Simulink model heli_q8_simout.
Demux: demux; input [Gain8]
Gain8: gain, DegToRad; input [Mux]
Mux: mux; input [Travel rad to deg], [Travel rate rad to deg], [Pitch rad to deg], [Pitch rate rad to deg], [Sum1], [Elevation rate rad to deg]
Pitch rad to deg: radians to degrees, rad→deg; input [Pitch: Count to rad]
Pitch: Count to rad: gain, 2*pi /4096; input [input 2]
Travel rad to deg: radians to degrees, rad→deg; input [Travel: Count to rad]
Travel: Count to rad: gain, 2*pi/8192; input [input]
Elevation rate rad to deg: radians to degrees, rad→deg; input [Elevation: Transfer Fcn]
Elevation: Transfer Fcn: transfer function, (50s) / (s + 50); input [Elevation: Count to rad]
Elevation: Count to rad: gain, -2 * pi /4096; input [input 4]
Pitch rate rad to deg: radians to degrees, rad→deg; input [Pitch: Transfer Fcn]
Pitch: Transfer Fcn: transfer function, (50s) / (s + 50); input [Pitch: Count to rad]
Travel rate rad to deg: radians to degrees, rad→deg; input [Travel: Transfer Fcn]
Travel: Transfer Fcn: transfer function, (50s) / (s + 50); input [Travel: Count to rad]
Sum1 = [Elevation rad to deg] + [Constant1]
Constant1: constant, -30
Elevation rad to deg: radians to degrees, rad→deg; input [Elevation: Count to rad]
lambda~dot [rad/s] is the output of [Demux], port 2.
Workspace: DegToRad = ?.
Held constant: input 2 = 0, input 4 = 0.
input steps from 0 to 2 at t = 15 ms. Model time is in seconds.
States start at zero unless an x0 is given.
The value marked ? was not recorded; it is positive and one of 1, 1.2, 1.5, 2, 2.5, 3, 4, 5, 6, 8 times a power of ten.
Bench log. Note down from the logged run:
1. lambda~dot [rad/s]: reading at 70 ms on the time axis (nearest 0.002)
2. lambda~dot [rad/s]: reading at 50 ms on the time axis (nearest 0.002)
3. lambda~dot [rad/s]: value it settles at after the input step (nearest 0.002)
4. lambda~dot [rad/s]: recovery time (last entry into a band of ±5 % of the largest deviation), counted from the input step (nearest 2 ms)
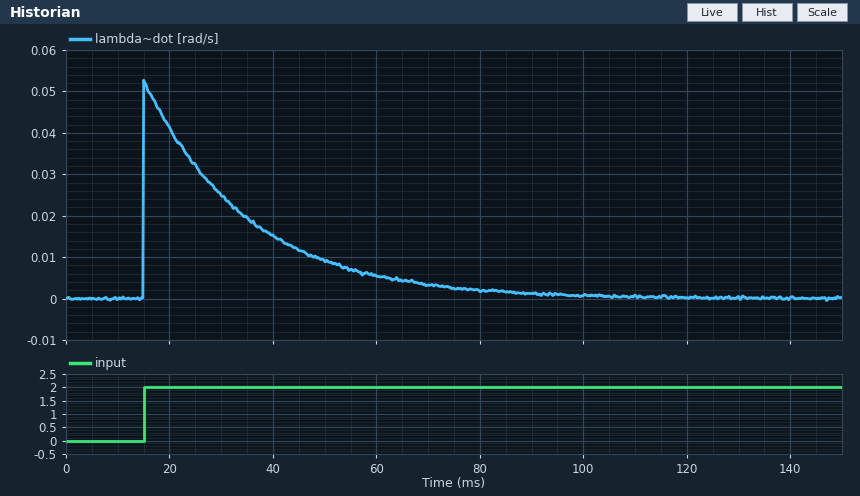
0.004
0.010
0.000
60 ms
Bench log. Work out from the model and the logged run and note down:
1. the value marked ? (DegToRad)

0.012
